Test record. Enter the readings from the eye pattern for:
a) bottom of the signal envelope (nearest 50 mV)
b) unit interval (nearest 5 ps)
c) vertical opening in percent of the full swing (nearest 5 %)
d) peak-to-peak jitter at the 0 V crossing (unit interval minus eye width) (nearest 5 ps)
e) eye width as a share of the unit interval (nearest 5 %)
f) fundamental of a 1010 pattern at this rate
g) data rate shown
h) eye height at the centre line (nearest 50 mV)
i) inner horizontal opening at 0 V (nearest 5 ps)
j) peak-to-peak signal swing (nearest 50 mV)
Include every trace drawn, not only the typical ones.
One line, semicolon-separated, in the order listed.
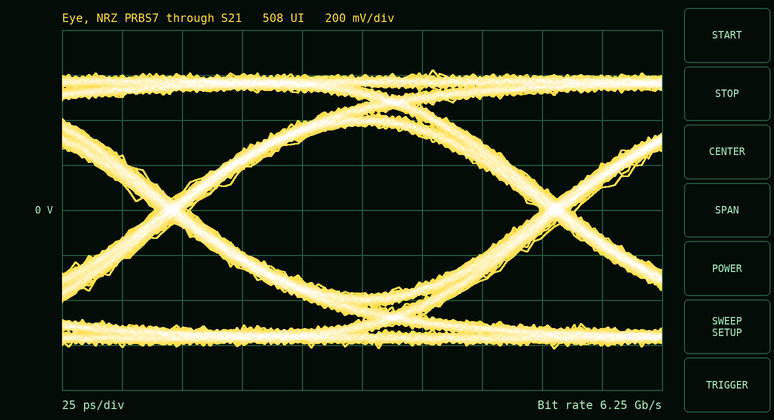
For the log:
-600 mV; 160 ps; 60 %; 15 ps; 90 %; 3.125 GHz; 6.25 Gb/s; 750 mV; 145 ps; 1.25 V
